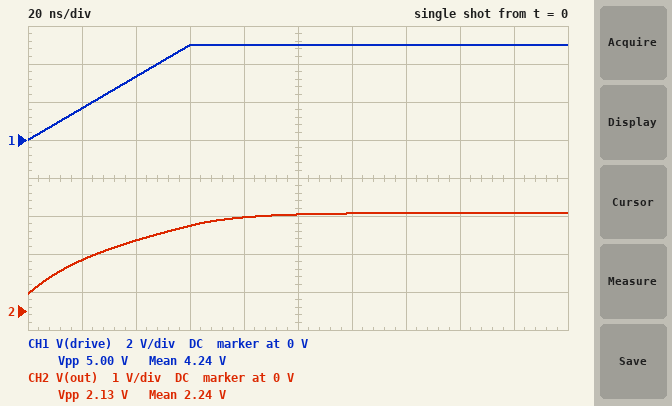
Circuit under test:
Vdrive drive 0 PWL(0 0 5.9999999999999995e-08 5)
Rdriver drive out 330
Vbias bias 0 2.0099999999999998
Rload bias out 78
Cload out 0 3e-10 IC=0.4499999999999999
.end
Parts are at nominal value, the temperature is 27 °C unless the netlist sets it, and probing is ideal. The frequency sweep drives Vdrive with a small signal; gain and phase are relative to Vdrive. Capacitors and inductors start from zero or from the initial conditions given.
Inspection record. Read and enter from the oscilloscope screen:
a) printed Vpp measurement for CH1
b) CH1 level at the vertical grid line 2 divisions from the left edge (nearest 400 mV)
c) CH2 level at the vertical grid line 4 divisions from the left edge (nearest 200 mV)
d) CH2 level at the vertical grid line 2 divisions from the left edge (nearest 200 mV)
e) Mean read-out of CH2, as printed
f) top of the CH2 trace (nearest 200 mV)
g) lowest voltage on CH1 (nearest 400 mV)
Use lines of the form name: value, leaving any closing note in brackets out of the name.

printed Vpp measurement for CH1: 5.00 V
CH1 level at the vertical grid line 2 divisions from the left edge: 3.2 V
CH2 level at the vertical grid line 4 divisions from the left edge: 2.4 V
CH2 level at the vertical grid line 2 divisions from the left edge: 1.8 V
Mean read-out of CH2, as printed: 2.24 V
top of the CH2 trace: 2.6 V
lowest voltage on CH1: 0 V
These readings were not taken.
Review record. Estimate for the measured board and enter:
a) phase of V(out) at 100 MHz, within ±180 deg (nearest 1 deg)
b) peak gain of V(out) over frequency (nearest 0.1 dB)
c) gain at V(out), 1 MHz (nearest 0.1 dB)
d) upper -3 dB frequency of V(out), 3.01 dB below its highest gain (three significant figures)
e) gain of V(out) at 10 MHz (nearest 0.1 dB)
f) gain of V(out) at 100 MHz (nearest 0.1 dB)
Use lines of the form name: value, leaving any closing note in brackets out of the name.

phase of V(out) at 100 MHz, within ±180 deg: -85 deg
peak gain of V(out) over frequency: -14.4 dB
gain at V(out), 1 MHz: -14.4 dB
upper -3 dB frequency of V(out), 3.01 dB below its highest gain: 8.41 MHz
gain of V(out) at 10 MHz: -18.2 dB
gain of V(out) at 100 MHz: -35.9 dB
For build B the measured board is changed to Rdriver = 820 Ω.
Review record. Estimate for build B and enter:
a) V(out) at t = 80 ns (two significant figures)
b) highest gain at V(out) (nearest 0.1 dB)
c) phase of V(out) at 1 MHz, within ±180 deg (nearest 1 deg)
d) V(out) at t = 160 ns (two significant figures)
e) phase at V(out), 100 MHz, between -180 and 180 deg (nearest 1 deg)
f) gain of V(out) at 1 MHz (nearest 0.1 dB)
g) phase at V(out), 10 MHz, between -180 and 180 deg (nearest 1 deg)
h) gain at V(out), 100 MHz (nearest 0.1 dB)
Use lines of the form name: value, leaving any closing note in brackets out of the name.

V(out) at t = 80 ns: 2.2 V
highest gain at V(out): -21.2 dB
phase of V(out) at 1 MHz, within ±180 deg: -8 deg
V(out) at t = 160 ns: 2.3 V
phase at V(out), 100 MHz, between -180 and 180 deg: -86 deg
gain of V(out) at 1 MHz: -21.3 dB
phase at V(out), 10 MHz, between -180 and 180 deg: -53 deg
gain at V(out), 100 MHz: -43.8 dB
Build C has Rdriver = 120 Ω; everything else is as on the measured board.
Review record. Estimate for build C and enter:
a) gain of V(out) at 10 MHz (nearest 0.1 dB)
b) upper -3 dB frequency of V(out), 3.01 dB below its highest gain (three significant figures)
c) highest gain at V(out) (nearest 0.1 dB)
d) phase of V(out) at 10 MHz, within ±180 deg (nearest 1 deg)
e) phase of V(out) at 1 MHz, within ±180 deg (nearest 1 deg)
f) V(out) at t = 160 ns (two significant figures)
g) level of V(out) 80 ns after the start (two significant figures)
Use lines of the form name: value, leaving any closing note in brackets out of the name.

gain of V(out) at 10 MHz: -10.6 dB
upper -3 dB frequency of V(out), 3.01 dB below its highest gain: 11.2 MHz
highest gain at V(out): -8.1 dB
phase of V(out) at 10 MHz, within ±180 deg: -42 deg
phase of V(out) at 1 MHz, within ±180 deg: -5 deg
V(out) at t = 160 ns: 3.2 V
level of V(out) 80 ns after the start: 3.1 V
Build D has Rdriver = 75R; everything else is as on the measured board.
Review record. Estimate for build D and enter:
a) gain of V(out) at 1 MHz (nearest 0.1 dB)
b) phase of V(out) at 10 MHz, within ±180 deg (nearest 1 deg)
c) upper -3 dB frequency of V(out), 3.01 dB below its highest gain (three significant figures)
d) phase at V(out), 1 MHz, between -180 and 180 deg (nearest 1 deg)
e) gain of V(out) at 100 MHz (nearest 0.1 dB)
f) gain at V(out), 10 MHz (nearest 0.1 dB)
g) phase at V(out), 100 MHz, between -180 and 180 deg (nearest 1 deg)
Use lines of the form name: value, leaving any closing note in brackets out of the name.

gain of V(out) at 1 MHz: -5.9 dB
phase of V(out) at 10 MHz, within ±180 deg: -36 deg
upper -3 dB frequency of V(out), 3.01 dB below its highest gain: 13.9 MHz
phase at V(out), 1 MHz, between -180 and 180 deg: -4 deg
gain of V(out) at 100 MHz: -23.1 dB
gain at V(out), 10 MHz: -7.7 dB
phase at V(out), 100 MHz, between -180 and 180 deg: -82 deg
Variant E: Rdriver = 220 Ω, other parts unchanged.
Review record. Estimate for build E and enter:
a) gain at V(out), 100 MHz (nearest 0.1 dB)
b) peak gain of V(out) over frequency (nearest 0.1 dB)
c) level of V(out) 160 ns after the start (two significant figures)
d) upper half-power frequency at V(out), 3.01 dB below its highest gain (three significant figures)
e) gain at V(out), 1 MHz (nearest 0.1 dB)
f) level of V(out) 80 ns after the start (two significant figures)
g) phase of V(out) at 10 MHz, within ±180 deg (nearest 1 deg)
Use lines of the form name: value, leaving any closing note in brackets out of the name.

gain at V(out), 100 MHz: -32.4 dB
peak gain of V(out) over frequency: -11.6 dB
level of V(out) 160 ns after the start: 2.8 V
upper half-power frequency at V(out), 3.01 dB below its highest gain: 9.21 MHz
gain at V(out), 1 MHz: -11.7 dB
level of V(out) 80 ns after the start: 2.7 V
phase of V(out) at 10 MHz, within ±180 deg: -47 deg
